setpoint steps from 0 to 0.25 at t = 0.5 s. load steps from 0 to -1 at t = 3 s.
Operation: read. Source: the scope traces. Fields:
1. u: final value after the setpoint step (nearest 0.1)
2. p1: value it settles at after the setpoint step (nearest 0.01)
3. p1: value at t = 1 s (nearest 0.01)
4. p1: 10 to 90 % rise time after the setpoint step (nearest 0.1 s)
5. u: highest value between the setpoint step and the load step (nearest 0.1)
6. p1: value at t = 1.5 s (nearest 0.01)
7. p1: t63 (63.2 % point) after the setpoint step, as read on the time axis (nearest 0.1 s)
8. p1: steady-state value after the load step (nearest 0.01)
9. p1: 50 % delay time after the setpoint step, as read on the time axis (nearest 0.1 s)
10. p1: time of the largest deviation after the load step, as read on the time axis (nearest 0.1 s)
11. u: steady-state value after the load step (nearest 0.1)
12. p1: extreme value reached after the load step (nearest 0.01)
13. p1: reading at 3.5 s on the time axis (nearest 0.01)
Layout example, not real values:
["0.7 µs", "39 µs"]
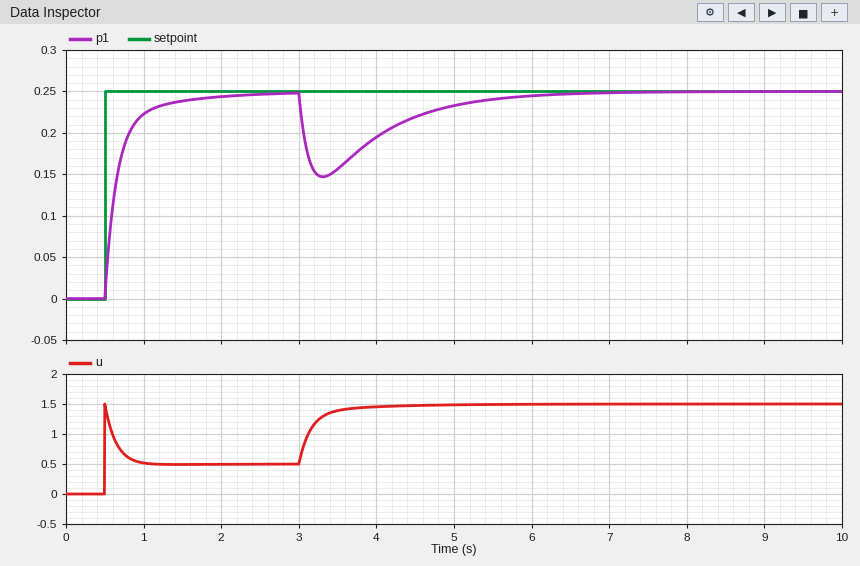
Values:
["0.5", "0.25", "0.22", "0.5 s", "1.5", "0.24", "0.7 s", "0.25", "0.6 s", "3.3 s", "1.5", "0.15", "0.16"]
